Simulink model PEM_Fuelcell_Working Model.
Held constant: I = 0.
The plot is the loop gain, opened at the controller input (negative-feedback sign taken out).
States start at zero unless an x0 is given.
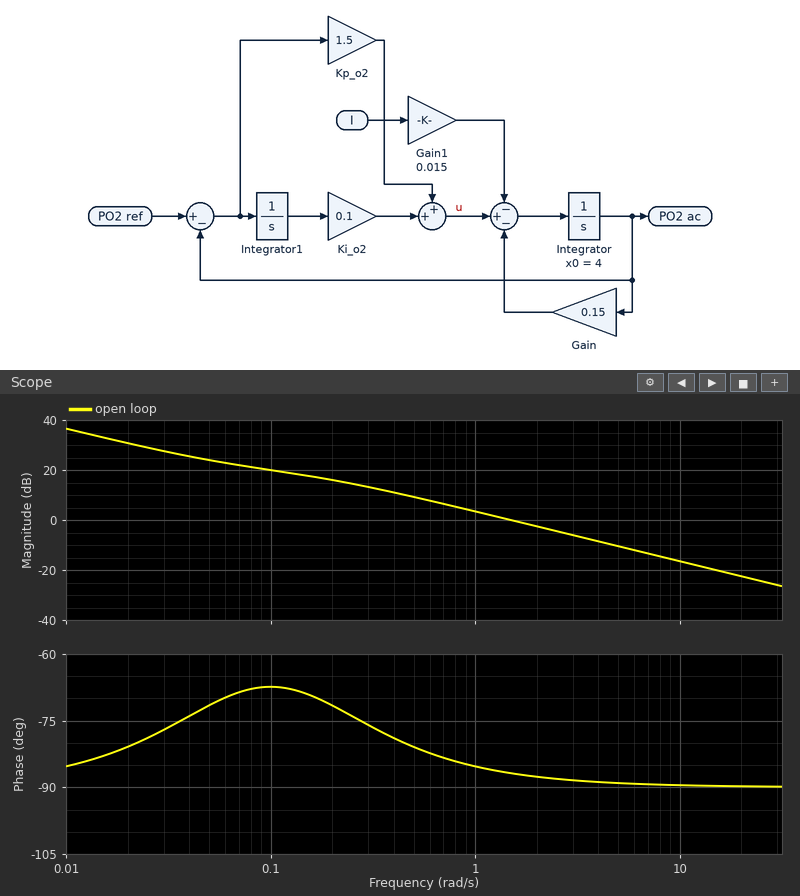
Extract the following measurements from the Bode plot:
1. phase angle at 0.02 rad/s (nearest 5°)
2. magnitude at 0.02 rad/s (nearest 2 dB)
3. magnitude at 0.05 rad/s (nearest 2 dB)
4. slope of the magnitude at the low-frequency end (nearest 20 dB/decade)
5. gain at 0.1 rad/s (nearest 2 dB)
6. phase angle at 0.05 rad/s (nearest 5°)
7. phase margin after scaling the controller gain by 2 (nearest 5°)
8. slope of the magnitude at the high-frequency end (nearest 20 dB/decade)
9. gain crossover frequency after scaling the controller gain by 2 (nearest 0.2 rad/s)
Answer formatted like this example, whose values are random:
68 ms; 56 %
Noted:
-80°; 30 dB; 24 dB; -20 dB/decade; 20 dB; -70°; 90°; -20 dB/decade; 3.0 rad/s
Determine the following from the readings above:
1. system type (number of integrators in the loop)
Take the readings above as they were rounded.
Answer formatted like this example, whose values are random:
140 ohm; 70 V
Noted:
1
